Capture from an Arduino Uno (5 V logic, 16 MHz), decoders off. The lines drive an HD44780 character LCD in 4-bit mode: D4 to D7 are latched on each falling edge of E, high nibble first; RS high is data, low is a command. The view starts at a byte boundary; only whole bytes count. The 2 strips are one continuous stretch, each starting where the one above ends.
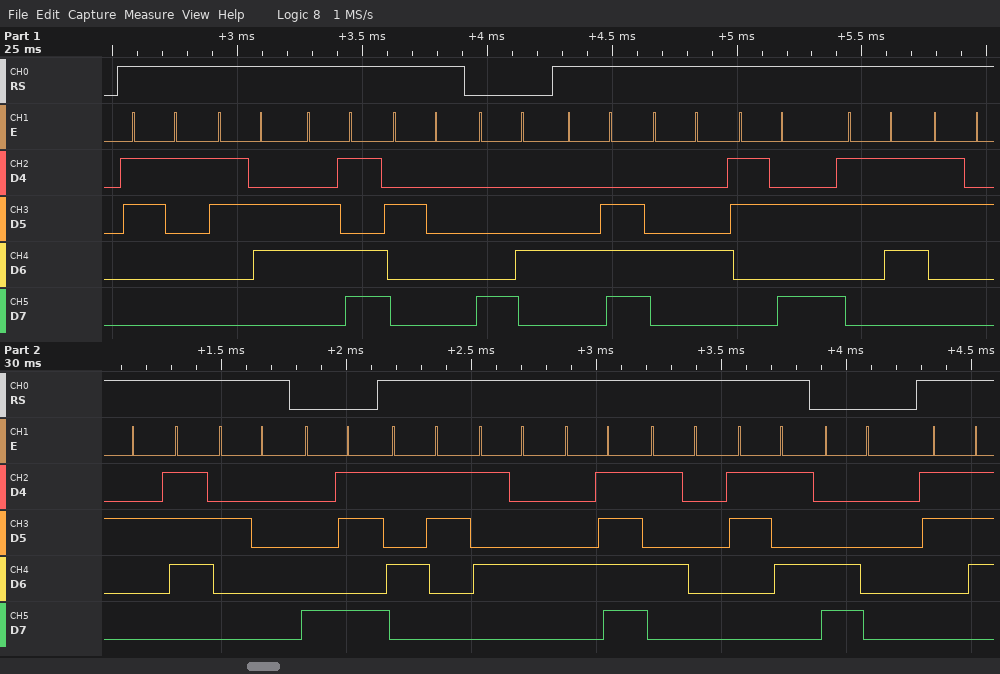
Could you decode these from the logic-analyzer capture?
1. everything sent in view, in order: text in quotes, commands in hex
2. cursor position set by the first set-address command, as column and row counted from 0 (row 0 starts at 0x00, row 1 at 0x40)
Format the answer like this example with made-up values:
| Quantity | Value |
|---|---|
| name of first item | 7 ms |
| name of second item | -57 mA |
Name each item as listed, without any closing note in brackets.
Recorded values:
| Quantity | Value |
|---|---|
| everything sent in view, in order: text in quotes, commands in hex | "16m " 0x84 "ND:72' " 0x8B "STOP5" 0xC0 "7" |
| cursor position set by the first set-address command, as column and row counted from 0 | column 4, row 0 |
